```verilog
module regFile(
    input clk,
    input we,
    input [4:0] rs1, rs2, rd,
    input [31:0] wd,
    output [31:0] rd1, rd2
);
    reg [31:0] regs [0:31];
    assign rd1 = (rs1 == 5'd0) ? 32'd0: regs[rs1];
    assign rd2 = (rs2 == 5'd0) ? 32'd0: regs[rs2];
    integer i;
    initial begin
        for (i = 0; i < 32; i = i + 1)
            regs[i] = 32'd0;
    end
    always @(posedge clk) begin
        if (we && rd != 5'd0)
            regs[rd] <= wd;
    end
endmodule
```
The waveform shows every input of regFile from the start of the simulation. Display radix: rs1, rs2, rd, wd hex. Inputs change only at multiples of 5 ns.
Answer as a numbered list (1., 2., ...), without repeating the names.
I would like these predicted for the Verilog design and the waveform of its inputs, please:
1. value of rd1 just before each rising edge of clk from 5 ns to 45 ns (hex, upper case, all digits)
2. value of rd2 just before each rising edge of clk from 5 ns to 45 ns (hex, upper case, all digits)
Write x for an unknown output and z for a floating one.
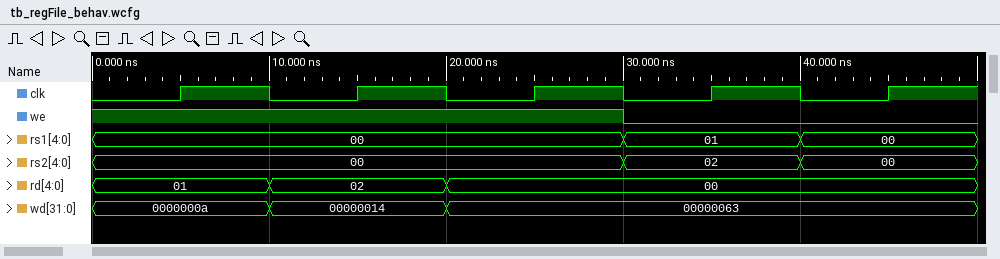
1. 00000000, 00000000, 00000000, 0000000A, 00000000
2. 00000000, 00000000, 00000000, 00000014, 00000000
